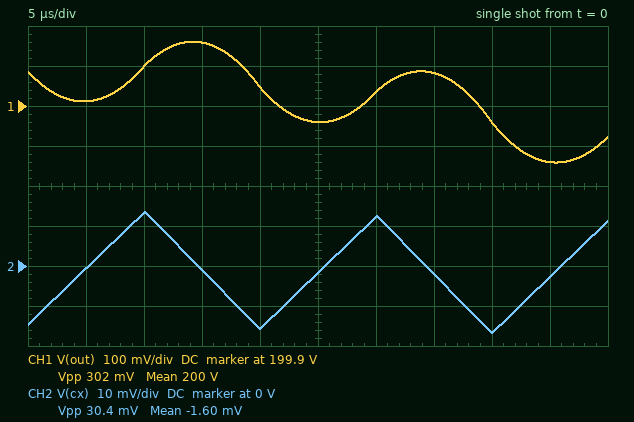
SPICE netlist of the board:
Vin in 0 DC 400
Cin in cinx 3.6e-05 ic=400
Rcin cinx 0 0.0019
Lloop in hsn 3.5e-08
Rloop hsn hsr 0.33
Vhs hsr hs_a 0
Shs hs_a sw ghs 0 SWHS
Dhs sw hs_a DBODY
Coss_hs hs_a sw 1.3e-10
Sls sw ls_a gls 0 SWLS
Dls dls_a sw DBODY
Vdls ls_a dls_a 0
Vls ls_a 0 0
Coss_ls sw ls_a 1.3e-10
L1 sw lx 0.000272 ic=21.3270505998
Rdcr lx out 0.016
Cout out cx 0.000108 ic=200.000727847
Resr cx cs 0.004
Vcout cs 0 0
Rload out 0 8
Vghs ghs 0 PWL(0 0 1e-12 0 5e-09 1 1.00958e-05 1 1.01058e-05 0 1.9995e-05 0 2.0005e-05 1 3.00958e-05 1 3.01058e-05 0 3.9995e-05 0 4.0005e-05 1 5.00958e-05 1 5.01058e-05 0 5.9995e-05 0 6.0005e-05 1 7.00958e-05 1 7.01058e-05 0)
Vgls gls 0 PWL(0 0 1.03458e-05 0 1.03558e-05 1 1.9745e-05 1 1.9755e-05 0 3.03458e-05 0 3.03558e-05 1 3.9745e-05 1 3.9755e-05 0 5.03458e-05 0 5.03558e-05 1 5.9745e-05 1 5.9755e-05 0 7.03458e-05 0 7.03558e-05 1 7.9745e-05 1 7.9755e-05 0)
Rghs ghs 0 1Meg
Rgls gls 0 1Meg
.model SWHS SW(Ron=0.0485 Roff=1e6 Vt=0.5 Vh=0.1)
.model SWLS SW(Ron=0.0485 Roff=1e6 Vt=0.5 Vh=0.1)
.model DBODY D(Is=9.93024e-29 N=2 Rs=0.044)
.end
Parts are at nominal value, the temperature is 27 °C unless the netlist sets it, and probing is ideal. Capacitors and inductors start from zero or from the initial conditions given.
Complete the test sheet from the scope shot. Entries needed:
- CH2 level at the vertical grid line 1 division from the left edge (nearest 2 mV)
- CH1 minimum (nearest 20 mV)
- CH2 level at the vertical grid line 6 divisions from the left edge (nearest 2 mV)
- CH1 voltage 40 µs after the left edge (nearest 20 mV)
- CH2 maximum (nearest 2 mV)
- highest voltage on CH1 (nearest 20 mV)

0 V
199.76 V
12 mV
199.86 V
14 mV
200.06 V
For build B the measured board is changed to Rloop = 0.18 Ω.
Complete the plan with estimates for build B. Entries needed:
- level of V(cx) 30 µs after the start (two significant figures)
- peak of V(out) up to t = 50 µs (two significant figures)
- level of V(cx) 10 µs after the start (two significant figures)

13 mV
200 V
14 mV
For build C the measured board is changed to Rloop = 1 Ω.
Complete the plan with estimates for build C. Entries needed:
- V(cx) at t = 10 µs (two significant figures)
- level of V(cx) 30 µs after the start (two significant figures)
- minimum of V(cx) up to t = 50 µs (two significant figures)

11 mV
7.6 mV
-21 mV
